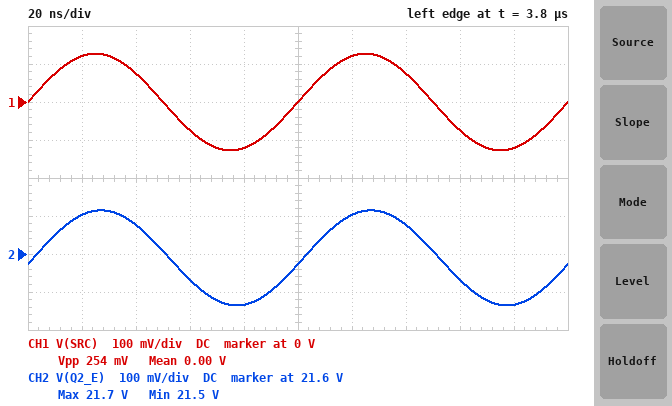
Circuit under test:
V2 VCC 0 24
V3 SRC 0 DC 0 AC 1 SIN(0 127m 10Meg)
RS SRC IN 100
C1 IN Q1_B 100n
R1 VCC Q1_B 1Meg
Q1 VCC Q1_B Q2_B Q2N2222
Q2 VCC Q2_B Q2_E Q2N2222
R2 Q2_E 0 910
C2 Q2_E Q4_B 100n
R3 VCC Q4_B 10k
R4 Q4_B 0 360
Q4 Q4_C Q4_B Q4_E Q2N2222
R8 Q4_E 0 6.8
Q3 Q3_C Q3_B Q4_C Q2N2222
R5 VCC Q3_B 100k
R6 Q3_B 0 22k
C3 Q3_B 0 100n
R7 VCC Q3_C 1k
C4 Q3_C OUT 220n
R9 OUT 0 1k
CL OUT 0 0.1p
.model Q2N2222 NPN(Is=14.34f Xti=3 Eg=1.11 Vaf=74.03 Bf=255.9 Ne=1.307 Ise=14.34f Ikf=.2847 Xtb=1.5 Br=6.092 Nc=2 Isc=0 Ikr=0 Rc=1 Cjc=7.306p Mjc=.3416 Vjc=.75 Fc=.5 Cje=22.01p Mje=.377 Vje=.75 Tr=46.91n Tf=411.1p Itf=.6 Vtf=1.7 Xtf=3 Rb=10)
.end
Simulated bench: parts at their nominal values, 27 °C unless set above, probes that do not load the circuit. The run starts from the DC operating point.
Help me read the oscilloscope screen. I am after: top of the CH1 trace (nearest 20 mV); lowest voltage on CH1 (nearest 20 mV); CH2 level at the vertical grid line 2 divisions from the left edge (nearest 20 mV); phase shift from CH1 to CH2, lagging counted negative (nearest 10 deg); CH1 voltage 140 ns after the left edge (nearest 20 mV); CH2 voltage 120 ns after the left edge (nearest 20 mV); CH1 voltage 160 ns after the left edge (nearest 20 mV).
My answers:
120 mV
-120 mV
21.68 V
-10 deg
80 mV
21.70 V
-80 mV
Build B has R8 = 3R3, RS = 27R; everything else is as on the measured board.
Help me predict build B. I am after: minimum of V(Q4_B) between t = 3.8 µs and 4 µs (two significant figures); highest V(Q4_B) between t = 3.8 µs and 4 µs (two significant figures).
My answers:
670 mV
920 mV
